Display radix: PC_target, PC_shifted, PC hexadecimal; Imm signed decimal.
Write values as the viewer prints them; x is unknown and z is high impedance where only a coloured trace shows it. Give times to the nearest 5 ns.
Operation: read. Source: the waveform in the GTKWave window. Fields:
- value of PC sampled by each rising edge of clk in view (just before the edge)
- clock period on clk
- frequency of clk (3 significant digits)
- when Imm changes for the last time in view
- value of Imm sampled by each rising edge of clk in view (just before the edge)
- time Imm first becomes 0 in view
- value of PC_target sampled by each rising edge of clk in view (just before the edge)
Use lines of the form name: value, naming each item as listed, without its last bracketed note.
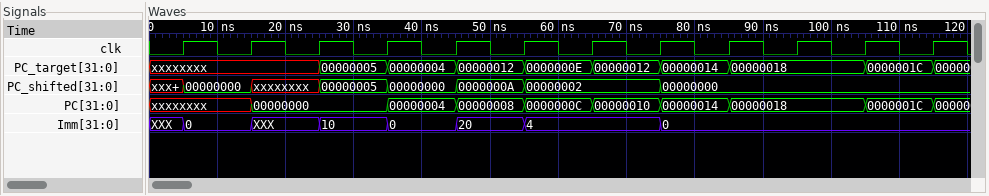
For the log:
value of PC sampled by each rising edge of clk in view: xxxxxxxx, xxxxxxxx, 00000000, 00000000, 00000004, 00000008, 0000000C, 00000010, 00000014, 00000018, 00000018, 0000001C
clock period on clk: 10 ns
frequency of clk: 100 MHz
when Imm changes for the last time in view: 75 ns
value of Imm sampled by each rising edge of clk in view: XXX, 0, XXX, 10, 0, 20, 4, 4, 0, 0, 0, 0
time Imm first becomes 0 in view: 5 ns
value of PC_target sampled by each rising edge of clk in view: xxxxxxxx, xxxxxxxx, xxxxxxxx, 00000005, 00000004, 00000012, 0000000E, 00000012, 00000014, 00000018, 00000018, 0000001C
